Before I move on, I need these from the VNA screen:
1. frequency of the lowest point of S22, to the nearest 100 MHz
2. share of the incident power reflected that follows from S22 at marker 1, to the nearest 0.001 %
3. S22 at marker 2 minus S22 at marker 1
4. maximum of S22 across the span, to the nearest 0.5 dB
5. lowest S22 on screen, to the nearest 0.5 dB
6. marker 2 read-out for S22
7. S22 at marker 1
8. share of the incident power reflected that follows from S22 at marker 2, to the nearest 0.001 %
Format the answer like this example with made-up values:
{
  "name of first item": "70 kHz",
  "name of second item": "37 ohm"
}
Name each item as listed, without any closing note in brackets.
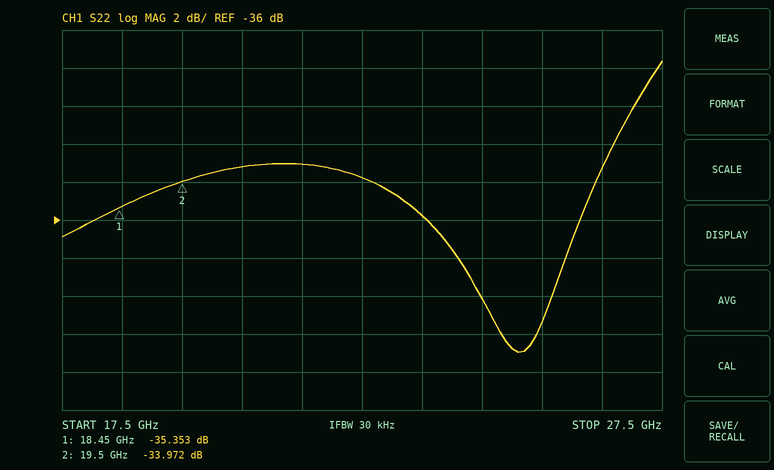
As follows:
{
  "frequency of the lowest point of S22, to the nearest 100 MHz": "25.1 GHz",
  "share of the incident power reflected that follows from S22 at marker 1, to the nearest 0.001 %": "0.029 %",
  "S22 at marker 2 minus S22 at marker 1": "1.381 dB",
  "maximum of S22 across the span, to the nearest 0.5 dB": "-27.5 dB",
  "lowest S22 on screen, to the nearest 0.5 dB": "-43.0 dB",
  "marker 2 read-out for S22": "-33.972 dB",
  "S22 at marker 1": "-35.353 dB",
  "share of the incident power reflected that follows from S22 at marker 2, to the nearest 0.001 %": "0.040 %"
}
